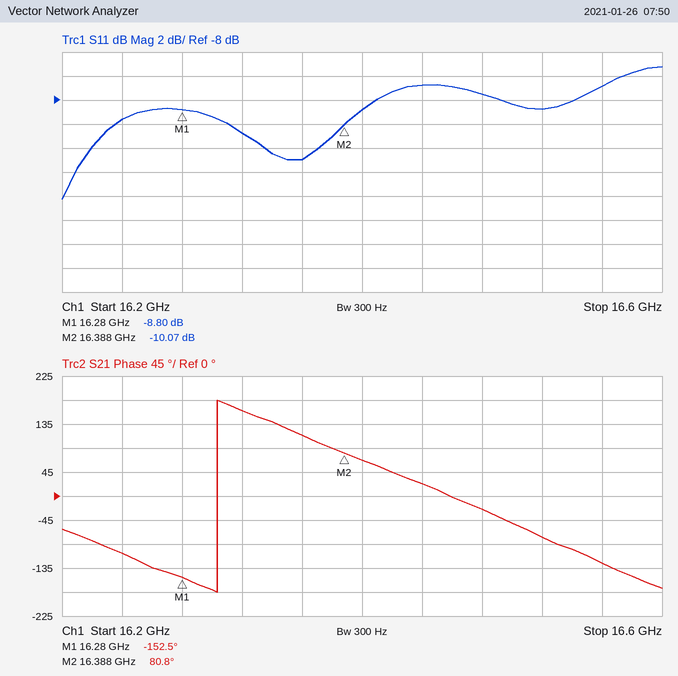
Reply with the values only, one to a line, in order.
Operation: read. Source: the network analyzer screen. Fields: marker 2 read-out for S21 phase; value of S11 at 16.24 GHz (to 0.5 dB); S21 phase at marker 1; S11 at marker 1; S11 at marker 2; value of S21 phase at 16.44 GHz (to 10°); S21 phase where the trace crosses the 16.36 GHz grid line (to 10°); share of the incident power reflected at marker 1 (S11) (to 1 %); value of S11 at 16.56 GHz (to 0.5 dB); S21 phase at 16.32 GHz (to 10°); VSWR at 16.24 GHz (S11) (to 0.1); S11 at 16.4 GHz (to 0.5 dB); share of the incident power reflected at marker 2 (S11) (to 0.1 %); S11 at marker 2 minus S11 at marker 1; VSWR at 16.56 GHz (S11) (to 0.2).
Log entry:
80.8°
-9.5 dB
-152.5°
-8.80 dB
-10.07 dB
20°
110°
13 %
-7.0 dB
160°
2.0
-9.0 dB
9.8 %
-1.27 dB
2.6
